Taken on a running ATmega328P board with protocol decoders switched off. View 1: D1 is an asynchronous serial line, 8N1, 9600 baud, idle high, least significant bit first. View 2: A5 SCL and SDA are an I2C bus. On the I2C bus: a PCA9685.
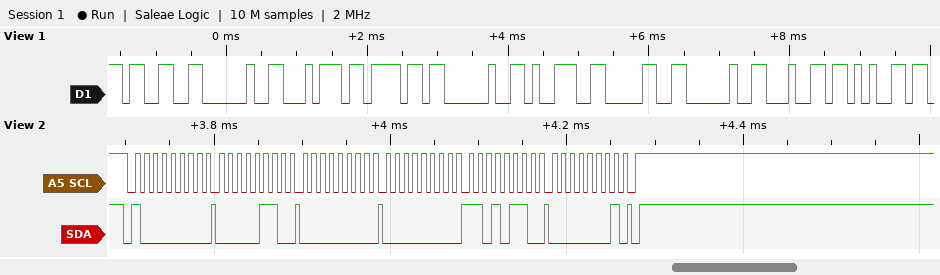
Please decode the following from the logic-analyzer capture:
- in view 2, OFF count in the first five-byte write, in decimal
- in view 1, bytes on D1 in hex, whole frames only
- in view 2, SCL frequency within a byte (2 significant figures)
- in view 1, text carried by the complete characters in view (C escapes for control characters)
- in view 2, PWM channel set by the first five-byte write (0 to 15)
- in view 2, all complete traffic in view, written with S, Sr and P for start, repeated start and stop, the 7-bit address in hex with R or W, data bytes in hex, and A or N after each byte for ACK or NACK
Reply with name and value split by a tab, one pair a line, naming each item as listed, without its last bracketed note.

in view 2, OFF count in the first five-byte write, in decimal	470
in view 1, bytes on D1 in hex, whole frames only	33 20 74 6F 20 39 30 20 64 65
in view 2, SCL frequency within a byte	100 kHz
in view 1, text carried by the complete characters in view	"3 to 90 de"
in view 2, PWM channel set by the first five-byte write	0
in view 2, all complete traffic in view, written with S, Sr and P for start, repeated start and stop, the 7-bit address in hex with R or W, data bytes in hex, and A or N after each byte for ACK or NACK	S 40W A 06 A 00 A 00 A D6 A 01 A P
